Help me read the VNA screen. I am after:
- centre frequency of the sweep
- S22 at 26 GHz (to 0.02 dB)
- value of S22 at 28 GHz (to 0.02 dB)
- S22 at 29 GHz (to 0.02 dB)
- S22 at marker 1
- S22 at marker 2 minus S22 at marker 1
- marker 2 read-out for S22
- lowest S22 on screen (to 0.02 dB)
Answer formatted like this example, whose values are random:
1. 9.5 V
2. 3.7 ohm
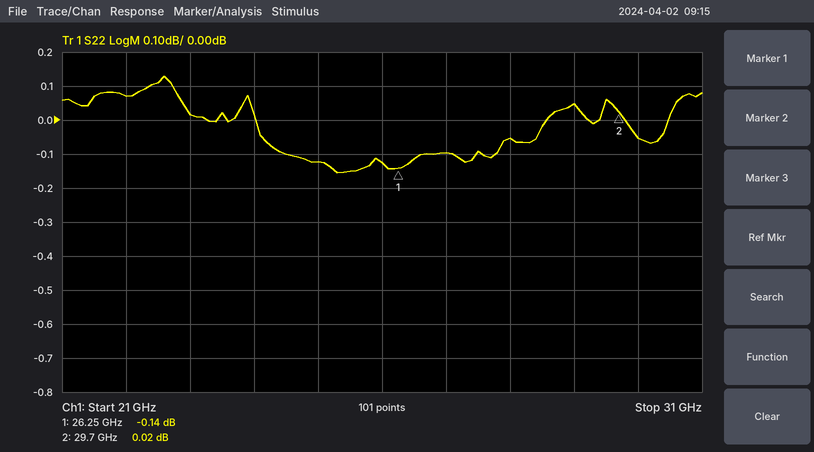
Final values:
1. 26 GHz
2. -0.12 dB
3. -0.06 dB
4. 0.04 dB
5. -0.14 dB
6. 0.16 dB
7. 0.02 dB
8. -0.16 dB
